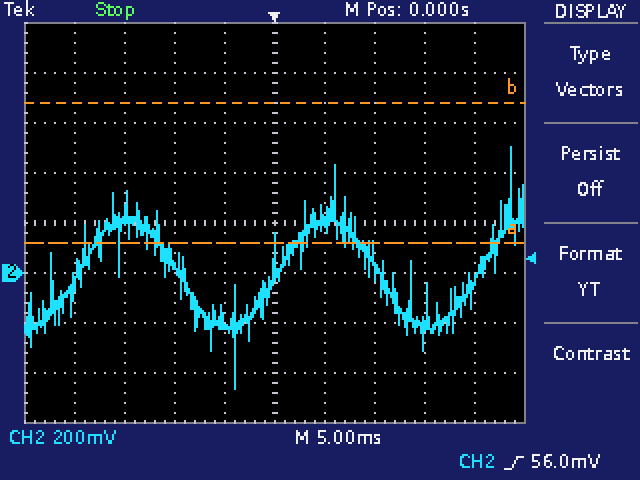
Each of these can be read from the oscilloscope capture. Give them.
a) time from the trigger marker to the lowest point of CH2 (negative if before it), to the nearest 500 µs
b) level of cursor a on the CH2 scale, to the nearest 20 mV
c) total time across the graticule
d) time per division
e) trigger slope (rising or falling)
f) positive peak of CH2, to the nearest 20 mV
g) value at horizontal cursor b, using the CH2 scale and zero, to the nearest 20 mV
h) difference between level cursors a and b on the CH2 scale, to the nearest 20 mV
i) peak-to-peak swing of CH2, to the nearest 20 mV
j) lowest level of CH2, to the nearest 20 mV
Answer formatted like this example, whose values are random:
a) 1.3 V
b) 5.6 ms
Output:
a) -4.0 ms
b) 120 mV
c) 50 ms
d) 5 ms
e) rising
f) 500 mV
g) 680 mV
h) 560 mV
i) 960 mV
j) -460 mV
